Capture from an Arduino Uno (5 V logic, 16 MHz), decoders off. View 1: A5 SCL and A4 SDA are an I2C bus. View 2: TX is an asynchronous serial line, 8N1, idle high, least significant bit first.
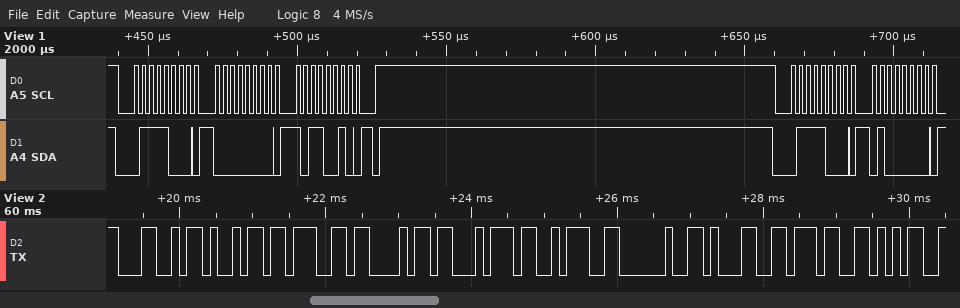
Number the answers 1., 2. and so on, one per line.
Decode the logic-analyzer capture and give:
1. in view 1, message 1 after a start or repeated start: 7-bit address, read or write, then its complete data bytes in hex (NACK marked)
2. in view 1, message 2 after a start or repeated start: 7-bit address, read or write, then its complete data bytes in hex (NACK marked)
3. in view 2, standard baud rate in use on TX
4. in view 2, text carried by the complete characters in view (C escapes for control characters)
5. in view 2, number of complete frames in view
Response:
1. 0x3C write: 00 B2
2. 0x3C write: 40
3. 9600 baud
4. "Light: 175"
5. 10
